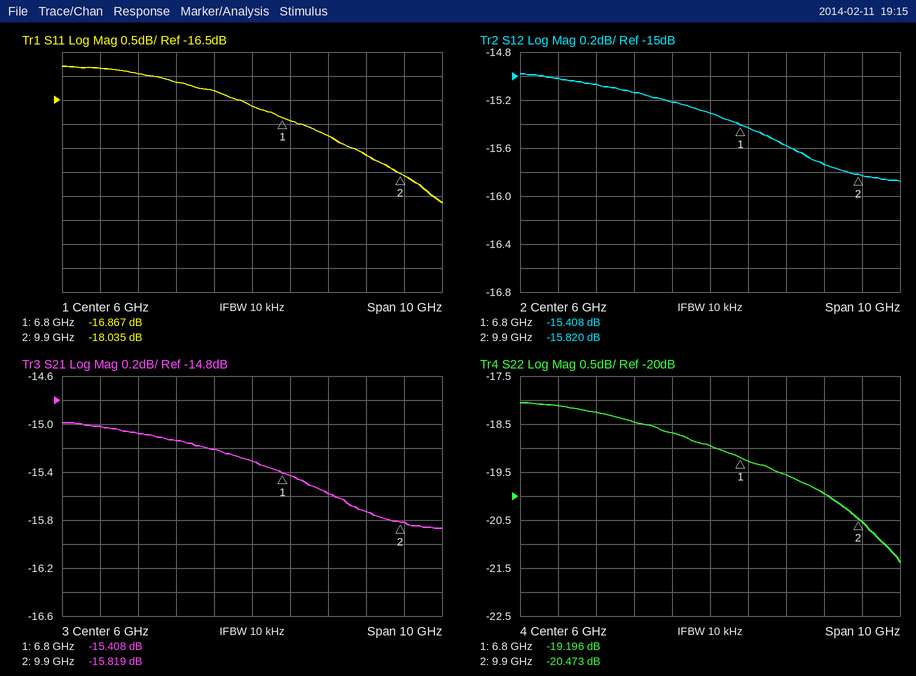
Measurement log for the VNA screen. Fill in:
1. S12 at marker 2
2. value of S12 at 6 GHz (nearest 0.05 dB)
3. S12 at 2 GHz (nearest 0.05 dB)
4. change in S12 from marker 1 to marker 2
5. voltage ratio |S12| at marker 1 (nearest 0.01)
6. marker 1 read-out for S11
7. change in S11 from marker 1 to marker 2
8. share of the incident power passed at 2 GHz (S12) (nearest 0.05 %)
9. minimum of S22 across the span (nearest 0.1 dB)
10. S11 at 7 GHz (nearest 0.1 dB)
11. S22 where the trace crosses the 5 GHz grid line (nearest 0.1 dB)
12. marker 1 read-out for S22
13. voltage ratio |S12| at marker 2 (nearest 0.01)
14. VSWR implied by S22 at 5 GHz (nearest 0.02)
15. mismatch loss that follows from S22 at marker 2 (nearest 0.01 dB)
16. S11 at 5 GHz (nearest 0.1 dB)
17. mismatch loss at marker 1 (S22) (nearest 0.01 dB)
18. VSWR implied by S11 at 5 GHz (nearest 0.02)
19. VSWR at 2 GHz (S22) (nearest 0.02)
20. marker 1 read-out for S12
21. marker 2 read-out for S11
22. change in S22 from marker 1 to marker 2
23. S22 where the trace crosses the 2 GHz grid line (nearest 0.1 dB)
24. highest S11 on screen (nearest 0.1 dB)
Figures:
-15.820 dB
-15.30 dB
-15.00 dB
-0.412 dB
0.17
-16.867 dB
-1.168 dB
3.15 %
-21.4 dB
-16.9 dB
-18.7 dB
-19.196 dB
0.16
1.26
0.04 dB
-16.3 dB
0.05 dB
1.36
1.28
-15.408 dB
-18.035 dB
-1.277 dB
-18.1 dB
-15.8 dB
